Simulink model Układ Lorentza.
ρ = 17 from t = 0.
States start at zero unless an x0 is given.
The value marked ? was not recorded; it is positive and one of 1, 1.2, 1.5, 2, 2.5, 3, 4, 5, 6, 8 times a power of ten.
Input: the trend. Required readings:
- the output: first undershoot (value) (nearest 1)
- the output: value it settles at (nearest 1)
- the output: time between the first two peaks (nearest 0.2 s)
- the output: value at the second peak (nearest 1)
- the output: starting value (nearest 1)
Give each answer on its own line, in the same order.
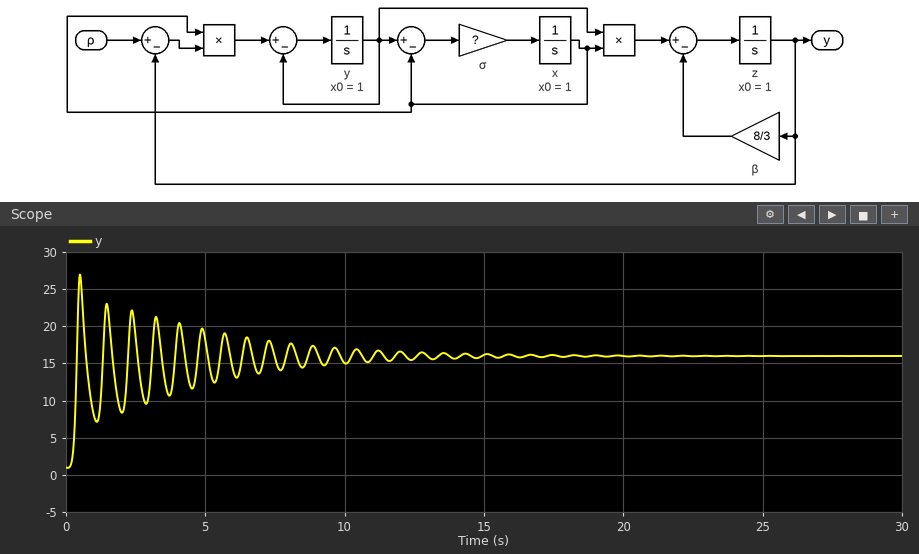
7
16
1.0 s
23
1
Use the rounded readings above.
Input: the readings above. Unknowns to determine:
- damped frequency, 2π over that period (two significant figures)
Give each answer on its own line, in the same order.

6.3 rad/s
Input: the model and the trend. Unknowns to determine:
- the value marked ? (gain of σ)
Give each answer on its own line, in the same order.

10
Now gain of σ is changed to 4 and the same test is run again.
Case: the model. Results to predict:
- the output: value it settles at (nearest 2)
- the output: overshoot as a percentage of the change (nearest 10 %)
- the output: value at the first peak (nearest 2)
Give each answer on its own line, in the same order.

16
70 %
26
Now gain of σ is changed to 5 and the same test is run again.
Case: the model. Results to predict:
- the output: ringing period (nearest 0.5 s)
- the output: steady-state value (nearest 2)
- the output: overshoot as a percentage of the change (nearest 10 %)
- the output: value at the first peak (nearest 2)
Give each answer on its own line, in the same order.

1.5 s
16
70 %
26
